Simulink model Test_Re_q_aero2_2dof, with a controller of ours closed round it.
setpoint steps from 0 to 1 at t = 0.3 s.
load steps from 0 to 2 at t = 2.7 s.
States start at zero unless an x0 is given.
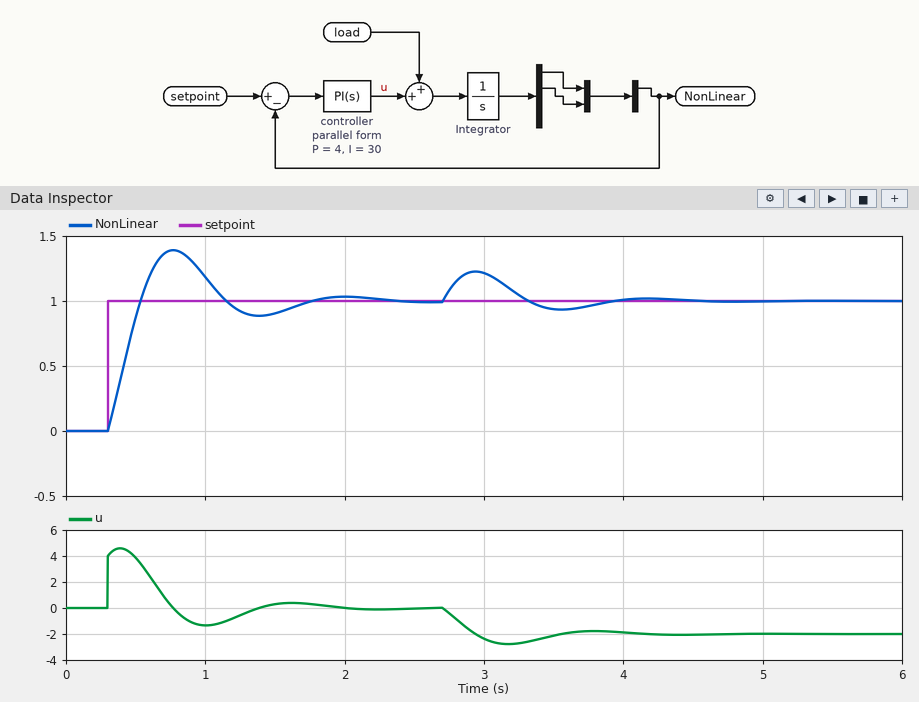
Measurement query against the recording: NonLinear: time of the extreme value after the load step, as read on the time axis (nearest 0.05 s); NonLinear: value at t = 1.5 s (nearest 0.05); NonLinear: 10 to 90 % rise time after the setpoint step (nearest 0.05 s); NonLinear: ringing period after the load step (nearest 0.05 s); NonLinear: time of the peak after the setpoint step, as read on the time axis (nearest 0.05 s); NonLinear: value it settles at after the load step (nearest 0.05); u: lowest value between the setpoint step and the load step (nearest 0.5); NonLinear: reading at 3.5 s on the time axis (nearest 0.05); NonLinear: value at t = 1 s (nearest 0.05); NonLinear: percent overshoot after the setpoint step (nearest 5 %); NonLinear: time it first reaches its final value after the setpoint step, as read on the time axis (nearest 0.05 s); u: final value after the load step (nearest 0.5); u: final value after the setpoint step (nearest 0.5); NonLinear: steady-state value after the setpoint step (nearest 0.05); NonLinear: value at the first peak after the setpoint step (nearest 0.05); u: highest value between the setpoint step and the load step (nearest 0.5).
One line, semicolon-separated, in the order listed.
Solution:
2.95 s; 0.90; 0.20 s; 1.25 s; 0.75 s; 1.00; -1.5; 0.95; 1.20; 40 %; 0.55 s; -2.0; 0.0; 1.00; 1.40; 4.5
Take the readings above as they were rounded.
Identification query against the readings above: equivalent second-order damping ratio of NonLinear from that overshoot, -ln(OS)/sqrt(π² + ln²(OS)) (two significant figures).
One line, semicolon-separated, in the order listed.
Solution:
0.28
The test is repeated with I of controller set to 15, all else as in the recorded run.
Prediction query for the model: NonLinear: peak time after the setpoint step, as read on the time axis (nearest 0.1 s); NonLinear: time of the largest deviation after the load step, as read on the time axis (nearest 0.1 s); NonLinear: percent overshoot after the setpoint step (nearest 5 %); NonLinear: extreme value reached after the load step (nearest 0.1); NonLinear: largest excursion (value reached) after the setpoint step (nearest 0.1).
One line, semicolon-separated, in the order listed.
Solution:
0.9 s; 3.0 s; 30 %; 1.3; 1.3
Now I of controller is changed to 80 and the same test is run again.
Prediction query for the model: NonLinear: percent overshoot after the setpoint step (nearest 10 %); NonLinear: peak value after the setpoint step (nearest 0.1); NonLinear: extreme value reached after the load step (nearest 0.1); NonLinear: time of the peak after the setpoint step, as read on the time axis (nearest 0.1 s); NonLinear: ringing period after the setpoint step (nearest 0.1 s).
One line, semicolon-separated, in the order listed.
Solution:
50 %; 1.5; 1.2; 0.6 s; 0.7 s
